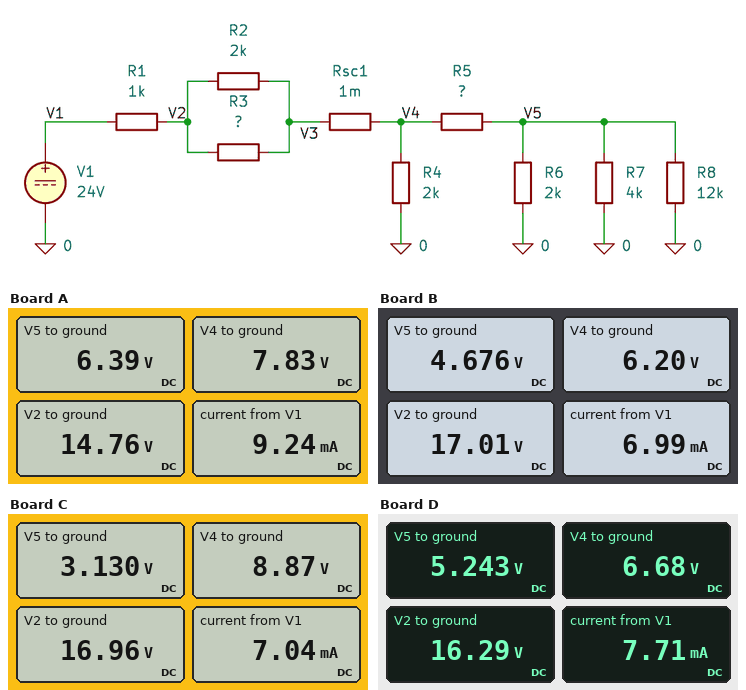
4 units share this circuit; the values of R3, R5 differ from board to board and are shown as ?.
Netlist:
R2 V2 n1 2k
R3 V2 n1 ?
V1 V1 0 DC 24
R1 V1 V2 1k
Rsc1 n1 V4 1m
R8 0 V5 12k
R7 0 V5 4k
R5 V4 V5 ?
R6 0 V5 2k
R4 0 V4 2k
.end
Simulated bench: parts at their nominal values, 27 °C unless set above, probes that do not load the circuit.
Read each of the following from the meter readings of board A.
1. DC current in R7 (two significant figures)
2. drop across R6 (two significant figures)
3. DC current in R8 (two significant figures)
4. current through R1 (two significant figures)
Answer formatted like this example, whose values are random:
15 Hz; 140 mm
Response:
1.6 mA; 6.4 V; 530 µA; 9.2 mA
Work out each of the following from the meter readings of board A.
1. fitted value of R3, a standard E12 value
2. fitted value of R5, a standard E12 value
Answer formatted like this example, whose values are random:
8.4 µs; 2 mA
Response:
1.2 kΩ; 270 Ω
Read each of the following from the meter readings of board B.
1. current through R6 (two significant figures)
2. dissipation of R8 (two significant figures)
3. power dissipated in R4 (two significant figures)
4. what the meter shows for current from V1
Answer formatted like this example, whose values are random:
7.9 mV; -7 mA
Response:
2.3 mA; 1.8 mW; 19 mW; 6.99 mA
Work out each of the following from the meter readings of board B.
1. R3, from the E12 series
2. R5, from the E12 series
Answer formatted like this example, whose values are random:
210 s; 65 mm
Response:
6.8 kΩ; 390 Ω
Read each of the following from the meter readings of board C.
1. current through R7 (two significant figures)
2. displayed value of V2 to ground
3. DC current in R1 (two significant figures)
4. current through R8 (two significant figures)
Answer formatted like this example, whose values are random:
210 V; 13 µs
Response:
780 µA; 16.96 V; 7.0 mA; 260 µA
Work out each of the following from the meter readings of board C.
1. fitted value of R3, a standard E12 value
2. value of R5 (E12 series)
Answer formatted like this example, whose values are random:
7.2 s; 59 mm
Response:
2.7 kΩ; 2.2 kΩ
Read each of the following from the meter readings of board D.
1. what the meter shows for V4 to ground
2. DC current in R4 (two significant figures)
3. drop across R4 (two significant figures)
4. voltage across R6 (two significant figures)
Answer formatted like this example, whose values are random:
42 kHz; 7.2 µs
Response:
6.68 V; 3.3 mA; 6.7 V; 5.2 V
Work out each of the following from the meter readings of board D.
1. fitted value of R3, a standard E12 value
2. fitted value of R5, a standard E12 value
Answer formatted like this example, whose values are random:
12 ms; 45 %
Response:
3.3 kΩ; 330 Ω
